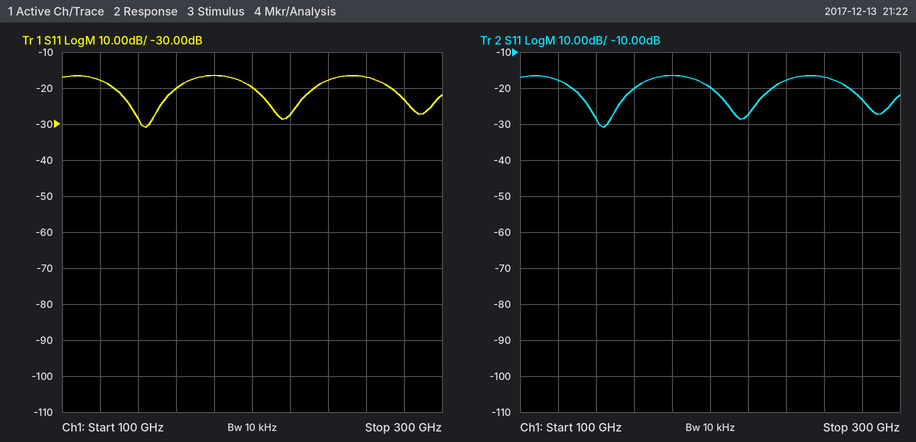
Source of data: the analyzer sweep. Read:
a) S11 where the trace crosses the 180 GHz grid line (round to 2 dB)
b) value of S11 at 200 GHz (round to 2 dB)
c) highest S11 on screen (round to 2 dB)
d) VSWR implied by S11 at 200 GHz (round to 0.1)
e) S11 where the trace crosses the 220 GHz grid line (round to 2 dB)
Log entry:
-16 dB
-20 dB
-16 dB
1.2
-28 dB
